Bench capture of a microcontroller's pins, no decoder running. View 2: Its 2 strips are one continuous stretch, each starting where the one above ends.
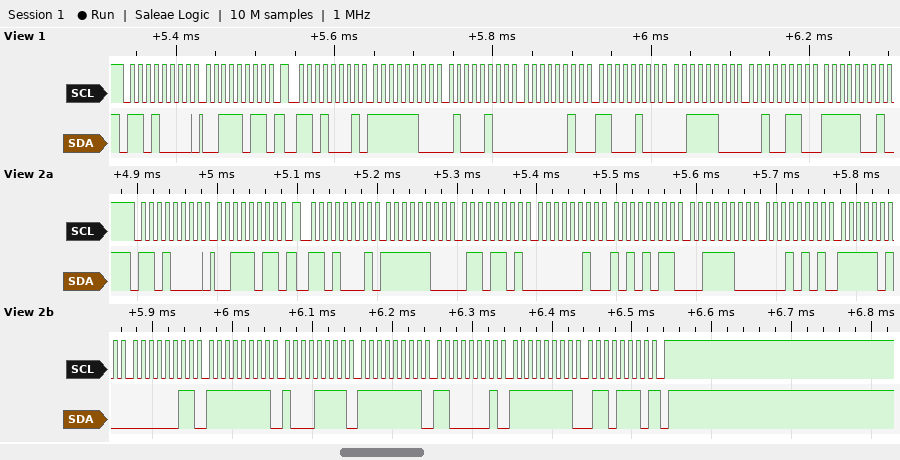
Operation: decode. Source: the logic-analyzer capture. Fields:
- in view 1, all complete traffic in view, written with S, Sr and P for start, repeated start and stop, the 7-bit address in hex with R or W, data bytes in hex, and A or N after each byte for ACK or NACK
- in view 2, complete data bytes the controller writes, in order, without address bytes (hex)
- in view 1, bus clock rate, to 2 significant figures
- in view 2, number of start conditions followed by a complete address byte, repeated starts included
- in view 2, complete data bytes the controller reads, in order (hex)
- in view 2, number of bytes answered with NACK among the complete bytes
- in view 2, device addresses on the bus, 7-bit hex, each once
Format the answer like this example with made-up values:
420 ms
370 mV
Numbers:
S 68W A 3B A Sr 68R A FC A 44 A 02 A C4 A 3C A 26 A F9 A
3B
100 kHz
2
FC 6D 02 AB 3C 15 FA 03 FF 8F FF C1 FF 6E
1
0x68
